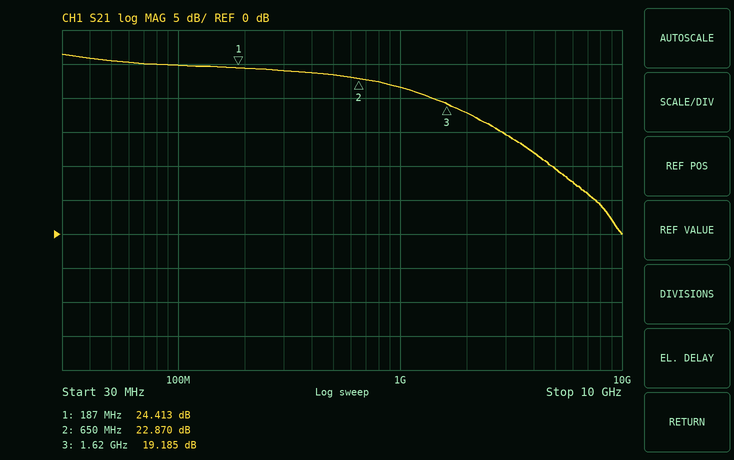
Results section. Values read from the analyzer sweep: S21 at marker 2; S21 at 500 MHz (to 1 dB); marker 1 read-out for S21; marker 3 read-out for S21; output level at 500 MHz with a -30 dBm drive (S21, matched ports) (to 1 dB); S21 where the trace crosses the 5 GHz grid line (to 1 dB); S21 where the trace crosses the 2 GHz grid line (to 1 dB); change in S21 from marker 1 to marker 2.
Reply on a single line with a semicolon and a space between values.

22.870 dB; 23 dB; 24.413 dB; 19.185 dB; -7 dBm; 10 dB; 18 dB; -1.543 dB
